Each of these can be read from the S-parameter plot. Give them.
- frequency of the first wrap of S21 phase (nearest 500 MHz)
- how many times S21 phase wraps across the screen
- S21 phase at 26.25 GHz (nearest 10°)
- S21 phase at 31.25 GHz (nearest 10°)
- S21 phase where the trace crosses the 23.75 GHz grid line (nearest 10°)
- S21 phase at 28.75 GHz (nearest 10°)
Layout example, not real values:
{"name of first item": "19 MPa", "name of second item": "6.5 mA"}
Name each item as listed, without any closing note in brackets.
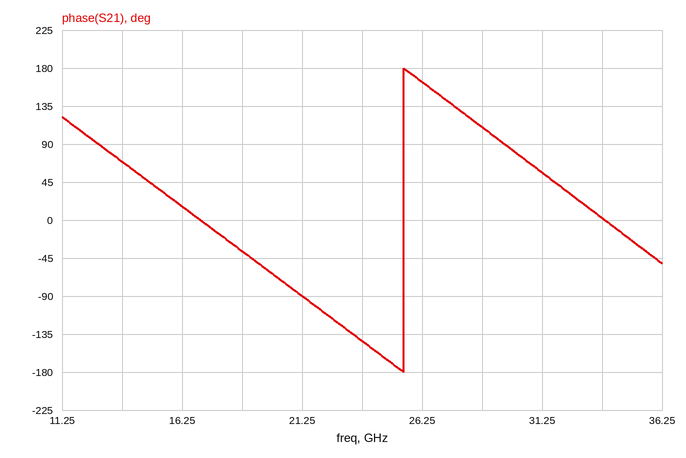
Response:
{"frequency of the first wrap of S21 phase": "25.5 GHz", "how many times S21 phase wraps across the screen": "1", "S21 phase at 26.25 GHz": "160°", "S21 phase at 31.25 GHz": "60°", "S21 phase where the trace crosses the 23.75 GHz grid line": "-140°", "S21 phase at 28.75 GHz": "110°"}
